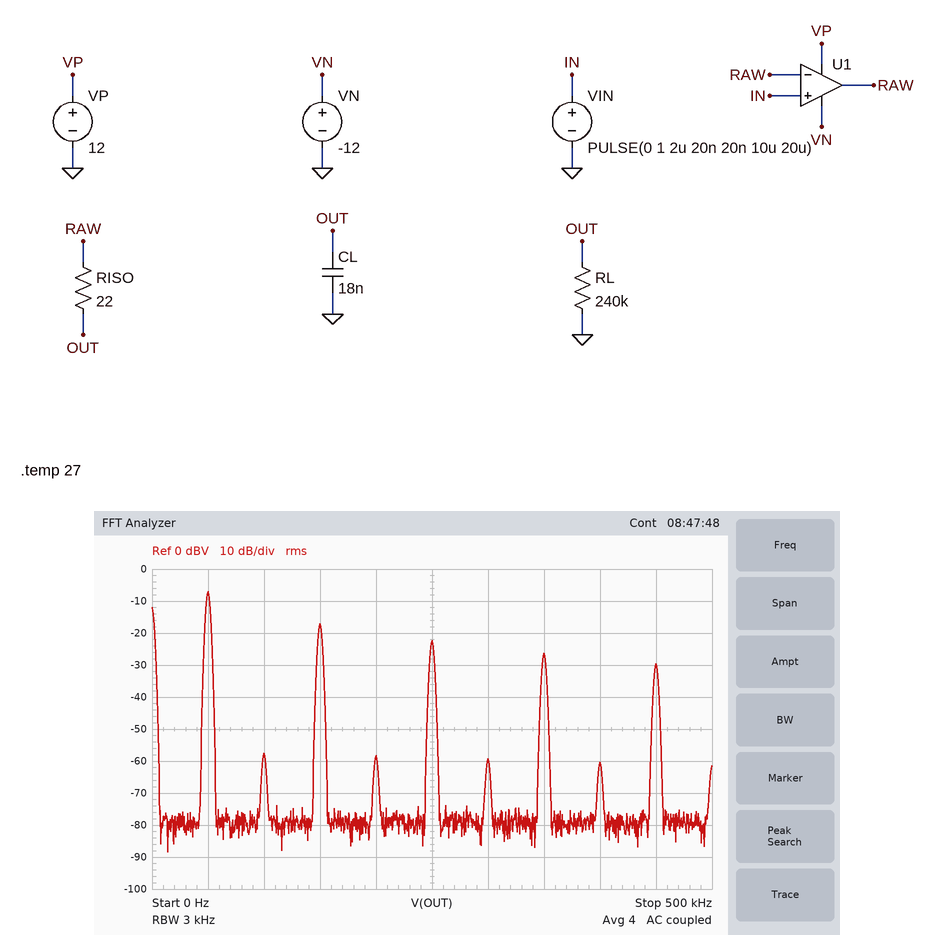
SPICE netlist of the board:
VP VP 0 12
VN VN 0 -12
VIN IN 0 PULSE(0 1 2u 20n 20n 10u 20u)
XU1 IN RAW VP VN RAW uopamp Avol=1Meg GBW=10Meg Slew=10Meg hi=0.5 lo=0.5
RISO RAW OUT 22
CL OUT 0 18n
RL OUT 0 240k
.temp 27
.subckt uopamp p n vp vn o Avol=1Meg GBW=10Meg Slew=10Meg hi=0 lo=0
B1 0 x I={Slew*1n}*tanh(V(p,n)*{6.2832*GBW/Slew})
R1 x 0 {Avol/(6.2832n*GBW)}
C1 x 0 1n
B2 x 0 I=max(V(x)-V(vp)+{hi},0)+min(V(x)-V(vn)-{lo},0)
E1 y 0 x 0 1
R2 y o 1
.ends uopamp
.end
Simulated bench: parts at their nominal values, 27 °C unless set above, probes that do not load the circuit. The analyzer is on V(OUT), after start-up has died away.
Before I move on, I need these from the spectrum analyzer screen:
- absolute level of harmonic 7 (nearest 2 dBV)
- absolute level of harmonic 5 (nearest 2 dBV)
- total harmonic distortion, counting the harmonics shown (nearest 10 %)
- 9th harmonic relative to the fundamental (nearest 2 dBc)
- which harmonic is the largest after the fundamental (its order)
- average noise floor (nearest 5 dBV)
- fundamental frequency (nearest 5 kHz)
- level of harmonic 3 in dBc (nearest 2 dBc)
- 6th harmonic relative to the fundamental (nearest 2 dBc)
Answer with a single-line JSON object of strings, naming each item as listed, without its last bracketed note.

{"absolute level of harmonic 7": "-26 dBV", "absolute level of harmonic 5": "-22 dBV", "total harmonic distortion, counting the harmonics shown": "40 %", "9th harmonic relative to the fundamental": "-22 dBc", "which harmonic is the largest after the fundamental": "3", "average noise floor": "-80 dBV", "fundamental frequency": "50 kHz", "level of harmonic 3 in dBc": "-10 dBc", "6th harmonic relative to the fundamental": "-52 dBc"}
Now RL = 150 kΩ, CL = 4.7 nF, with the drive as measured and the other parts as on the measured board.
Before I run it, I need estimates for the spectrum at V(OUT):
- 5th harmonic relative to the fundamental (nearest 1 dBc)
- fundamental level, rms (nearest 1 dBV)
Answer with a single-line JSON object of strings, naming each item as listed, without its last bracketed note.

{"5th harmonic relative to the fundamental": "-14 dBc", "fundamental level, rms": "-7 dBV"}
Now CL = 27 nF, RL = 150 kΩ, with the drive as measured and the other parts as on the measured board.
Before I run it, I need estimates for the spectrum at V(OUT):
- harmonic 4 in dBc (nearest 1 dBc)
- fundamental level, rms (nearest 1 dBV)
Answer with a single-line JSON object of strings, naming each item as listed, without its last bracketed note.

{"harmonic 4 in dBc": "-52 dBc", "fundamental level, rms": "-7 dBV"}
